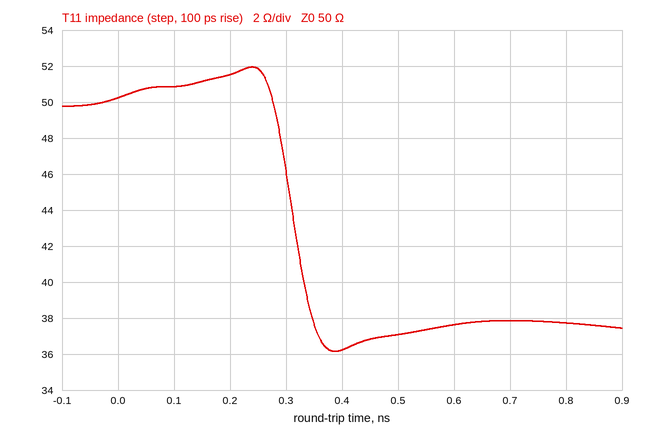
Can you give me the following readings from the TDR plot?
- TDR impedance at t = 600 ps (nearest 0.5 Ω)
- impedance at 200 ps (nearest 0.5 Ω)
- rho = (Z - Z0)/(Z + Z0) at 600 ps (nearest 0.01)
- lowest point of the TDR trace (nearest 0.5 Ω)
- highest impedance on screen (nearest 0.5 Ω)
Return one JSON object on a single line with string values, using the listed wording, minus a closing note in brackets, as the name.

{"TDR impedance at t = 600 ps": "37.5 Ω", "impedance at 200 ps": "51.5 Ω", "rho = (Z - Z0)/(Z + Z0) at 600 ps": "-0.14", "lowest point of the TDR trace": "36.0 Ω", "highest impedance on screen": "52.0 Ω"}
